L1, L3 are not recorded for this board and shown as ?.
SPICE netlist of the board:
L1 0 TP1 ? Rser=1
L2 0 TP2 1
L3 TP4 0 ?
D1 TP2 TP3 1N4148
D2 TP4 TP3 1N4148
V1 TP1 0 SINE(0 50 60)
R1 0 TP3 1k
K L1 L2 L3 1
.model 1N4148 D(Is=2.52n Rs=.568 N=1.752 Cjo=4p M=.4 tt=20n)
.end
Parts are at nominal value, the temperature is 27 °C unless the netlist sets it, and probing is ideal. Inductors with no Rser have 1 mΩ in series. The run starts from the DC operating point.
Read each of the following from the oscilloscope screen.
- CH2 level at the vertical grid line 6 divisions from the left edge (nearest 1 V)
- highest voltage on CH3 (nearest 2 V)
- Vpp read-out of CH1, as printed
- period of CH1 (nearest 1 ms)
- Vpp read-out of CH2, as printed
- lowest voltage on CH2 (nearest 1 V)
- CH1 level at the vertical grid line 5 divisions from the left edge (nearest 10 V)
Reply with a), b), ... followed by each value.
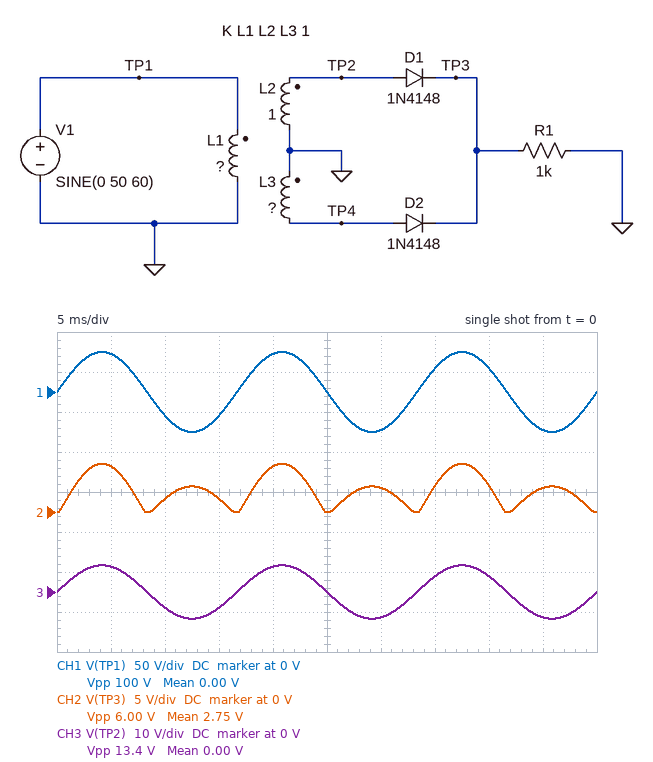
a) 3 V
b) 6 V
c) 100 V
d) 17 ms
e) 6.00 V
f) 0 V
g) 0 V
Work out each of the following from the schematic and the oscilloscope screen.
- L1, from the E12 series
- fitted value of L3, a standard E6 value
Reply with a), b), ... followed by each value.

a) 56 H
b) 330 mH
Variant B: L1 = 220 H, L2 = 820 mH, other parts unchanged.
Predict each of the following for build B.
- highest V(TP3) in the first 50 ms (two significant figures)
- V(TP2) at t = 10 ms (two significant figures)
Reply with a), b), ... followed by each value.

a) 2.4 V
b) -1.8 V
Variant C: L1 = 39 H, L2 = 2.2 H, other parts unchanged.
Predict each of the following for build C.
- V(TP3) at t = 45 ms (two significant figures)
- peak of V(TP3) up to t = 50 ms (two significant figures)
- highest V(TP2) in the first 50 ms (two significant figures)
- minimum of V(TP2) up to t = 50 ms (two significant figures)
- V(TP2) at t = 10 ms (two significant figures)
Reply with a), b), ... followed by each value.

a) 3.7 V
b) 11 V
c) 12 V
d) -12 V
e) -7.0 V
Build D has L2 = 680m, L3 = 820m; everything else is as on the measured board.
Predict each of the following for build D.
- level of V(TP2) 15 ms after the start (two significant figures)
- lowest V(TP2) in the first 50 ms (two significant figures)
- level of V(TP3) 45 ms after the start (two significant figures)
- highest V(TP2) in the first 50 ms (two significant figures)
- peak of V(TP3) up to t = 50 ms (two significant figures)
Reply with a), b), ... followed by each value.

a) -3.2 V
b) -5.5 V
c) 5.1 V
d) 5.5 V
e) 5.4 V
